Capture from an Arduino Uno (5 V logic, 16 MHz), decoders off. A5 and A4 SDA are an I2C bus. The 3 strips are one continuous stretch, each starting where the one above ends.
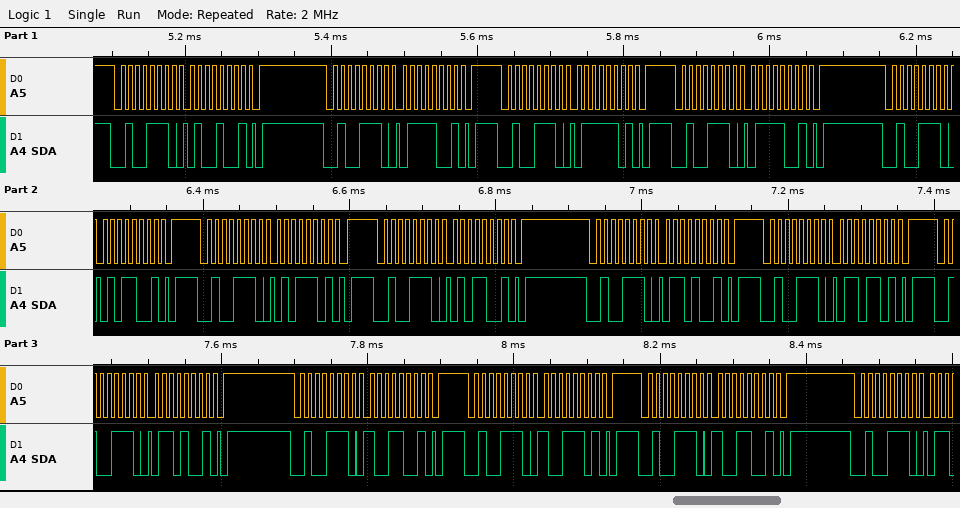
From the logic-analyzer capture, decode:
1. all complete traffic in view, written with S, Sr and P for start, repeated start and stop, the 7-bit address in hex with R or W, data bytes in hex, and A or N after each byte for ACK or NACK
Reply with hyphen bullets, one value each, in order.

- S 27W A 49 A P S 27W A 79 A P S 27W A 7D A P S 27W A 79 A P S 27W A 59 A P S 27W A 5D A P S 27W A 59 A P S 27W A 69 A P S 27W A 6D A P S 27W A 69 A P S 27W A 99 A P S 27W A 9D A P S 27W A 99 A P S 27W A
